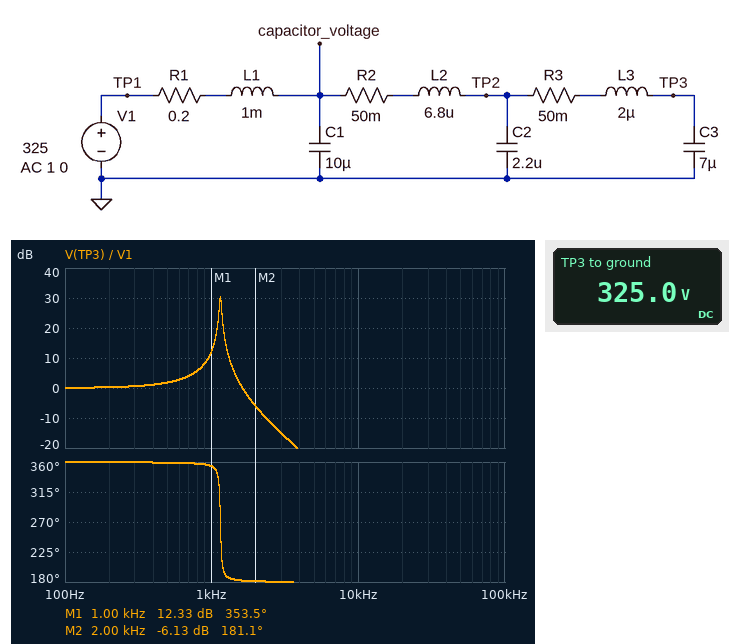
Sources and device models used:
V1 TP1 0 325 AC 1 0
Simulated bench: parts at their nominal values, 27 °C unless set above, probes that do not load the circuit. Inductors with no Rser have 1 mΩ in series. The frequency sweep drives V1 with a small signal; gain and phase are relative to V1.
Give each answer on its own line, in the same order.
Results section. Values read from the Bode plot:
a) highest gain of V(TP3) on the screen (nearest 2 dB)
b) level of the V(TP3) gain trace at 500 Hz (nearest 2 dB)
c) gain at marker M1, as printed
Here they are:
30 dB
2 dB
12.33 dB
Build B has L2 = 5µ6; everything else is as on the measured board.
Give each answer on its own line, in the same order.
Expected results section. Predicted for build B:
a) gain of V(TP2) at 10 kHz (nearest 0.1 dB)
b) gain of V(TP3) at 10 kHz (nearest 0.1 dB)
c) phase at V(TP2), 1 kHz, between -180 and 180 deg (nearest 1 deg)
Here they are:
-36.7 dB
-36.2 dB
-6 deg
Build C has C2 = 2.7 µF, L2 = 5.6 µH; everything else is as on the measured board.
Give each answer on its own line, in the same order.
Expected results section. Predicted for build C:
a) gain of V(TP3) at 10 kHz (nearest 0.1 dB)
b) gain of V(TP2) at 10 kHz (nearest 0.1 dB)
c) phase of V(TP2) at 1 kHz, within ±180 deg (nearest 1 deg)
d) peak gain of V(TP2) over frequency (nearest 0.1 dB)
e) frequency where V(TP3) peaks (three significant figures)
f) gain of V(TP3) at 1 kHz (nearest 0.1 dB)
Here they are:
-36.4 dB
-36.9 dB
-7 deg
30.2 dB
1.13 kHz
13.1 dB
